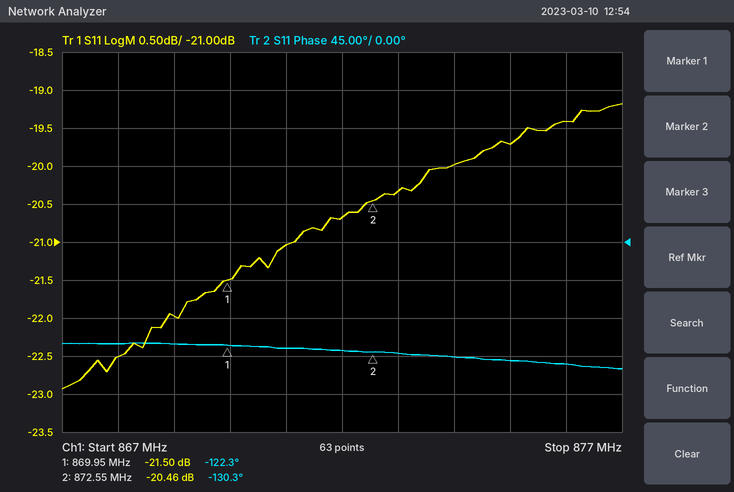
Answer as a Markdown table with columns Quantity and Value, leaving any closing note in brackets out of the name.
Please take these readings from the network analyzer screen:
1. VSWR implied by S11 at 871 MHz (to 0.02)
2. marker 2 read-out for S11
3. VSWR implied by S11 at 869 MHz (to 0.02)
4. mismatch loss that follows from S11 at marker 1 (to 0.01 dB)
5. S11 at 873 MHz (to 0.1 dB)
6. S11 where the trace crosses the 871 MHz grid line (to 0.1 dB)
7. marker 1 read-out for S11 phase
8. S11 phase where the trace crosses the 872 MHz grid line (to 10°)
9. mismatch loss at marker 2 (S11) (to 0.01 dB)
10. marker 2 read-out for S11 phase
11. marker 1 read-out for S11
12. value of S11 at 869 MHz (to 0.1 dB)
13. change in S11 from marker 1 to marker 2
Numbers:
| Quantity | Value |
|---|---|
| VSWR implied by S11 at 871 MHz | 1.20 |
| marker 2 read-out for S11 | -20.46 dB |
| VSWR implied by S11 at 869 MHz | 1.18 |
| mismatch loss that follows from S11 at marker 1 | 0.03 dB |
| S11 at 873 MHz | -20.3 dB |
| S11 where the trace crosses the 871 MHz grid line | -21.0 dB |
| marker 1 read-out for S11 phase | -122.3° |
| S11 phase where the trace crosses the 872 MHz grid line | -130° |
| mismatch loss at marker 2 (S11) | 0.04 dB |
| marker 2 read-out for S11 phase | -130.3° |
| marker 1 read-out for S11 | -21.50 dB |
| value of S11 at 869 MHz | -22.0 dB |
| change in S11 from marker 1 to marker 2 | 1.04 dB |
